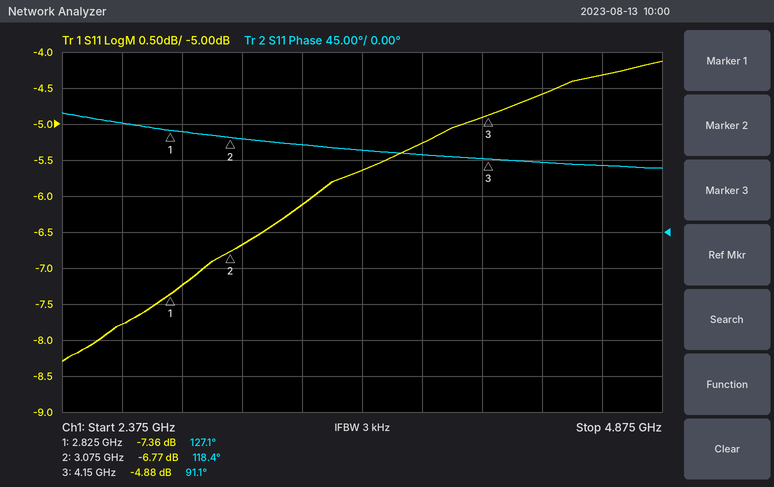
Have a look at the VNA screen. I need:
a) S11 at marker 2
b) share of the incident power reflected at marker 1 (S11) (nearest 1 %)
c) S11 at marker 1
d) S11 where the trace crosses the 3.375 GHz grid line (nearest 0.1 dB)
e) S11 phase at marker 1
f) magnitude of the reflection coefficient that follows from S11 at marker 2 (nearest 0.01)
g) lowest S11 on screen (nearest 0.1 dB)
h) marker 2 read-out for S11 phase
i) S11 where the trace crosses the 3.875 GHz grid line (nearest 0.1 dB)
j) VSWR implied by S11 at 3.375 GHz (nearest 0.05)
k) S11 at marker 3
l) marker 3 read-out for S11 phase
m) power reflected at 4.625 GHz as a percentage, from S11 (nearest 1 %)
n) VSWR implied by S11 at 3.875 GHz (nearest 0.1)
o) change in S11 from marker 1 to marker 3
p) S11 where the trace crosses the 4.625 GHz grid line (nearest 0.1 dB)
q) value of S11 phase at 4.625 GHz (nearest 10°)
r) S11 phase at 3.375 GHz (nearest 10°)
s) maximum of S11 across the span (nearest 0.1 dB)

-6.77 dB
18 %
-7.36 dB
-6.1 dB
127.1°
0.46
-8.3 dB
118.4°
-5.3 dB
2.95
-4.88 dB
91.1°
37 %
3.4
2.48 dB
-4.3 dB
80°
110°
-4.1 dB
